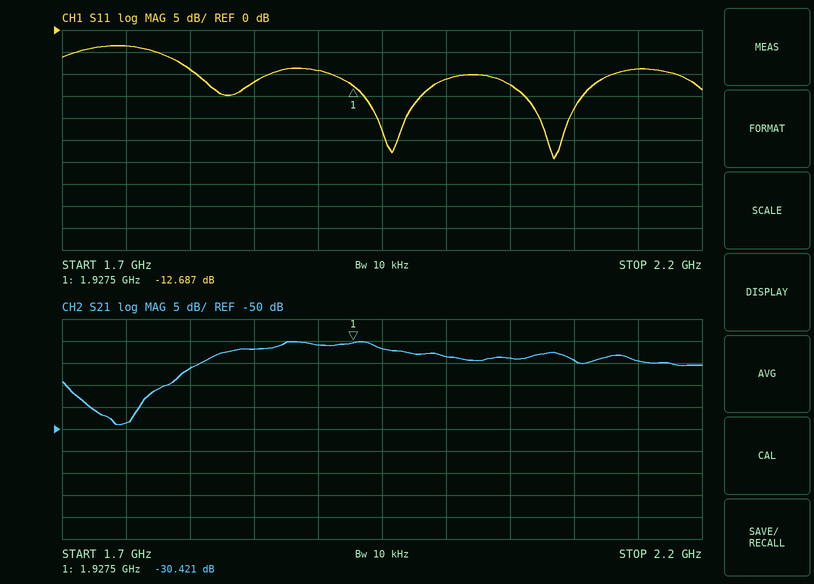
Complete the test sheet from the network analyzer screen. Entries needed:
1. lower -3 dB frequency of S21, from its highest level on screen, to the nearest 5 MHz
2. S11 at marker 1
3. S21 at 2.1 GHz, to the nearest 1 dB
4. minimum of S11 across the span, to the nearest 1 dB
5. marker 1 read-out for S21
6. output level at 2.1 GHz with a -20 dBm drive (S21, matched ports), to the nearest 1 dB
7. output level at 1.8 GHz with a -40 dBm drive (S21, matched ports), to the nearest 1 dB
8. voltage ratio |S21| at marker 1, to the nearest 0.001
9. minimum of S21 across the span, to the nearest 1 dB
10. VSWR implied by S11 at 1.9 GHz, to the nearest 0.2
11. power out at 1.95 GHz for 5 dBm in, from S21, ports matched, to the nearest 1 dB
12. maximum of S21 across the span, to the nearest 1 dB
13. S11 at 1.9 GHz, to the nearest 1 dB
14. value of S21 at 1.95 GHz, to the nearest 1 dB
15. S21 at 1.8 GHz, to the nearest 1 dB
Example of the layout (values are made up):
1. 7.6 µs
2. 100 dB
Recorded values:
1. 1.820 GHz
2. -12.687 dB
3. -34 dB
4. -29 dB
5. -30.421 dB
6. -54 dBm
7. -76 dBm
8. 0.030
9. -49 dB
10. 2.0
11. -27 dBm
12. -30 dB
13. -9 dB
14. -32 dB
15. -36 dB
